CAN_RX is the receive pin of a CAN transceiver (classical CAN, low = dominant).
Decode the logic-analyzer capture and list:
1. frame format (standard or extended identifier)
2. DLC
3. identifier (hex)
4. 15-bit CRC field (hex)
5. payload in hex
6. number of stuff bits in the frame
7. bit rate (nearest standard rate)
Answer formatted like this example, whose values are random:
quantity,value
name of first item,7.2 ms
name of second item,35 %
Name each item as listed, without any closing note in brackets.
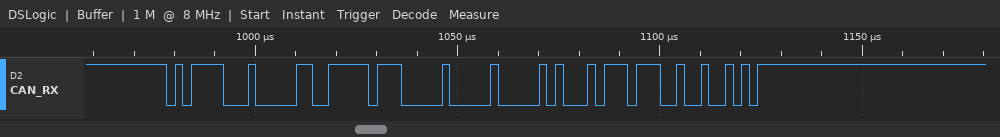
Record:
quantity,value
frame format,standard
DLC,4
identifier,0x5E2
15-bit CRC field,0x5C92
payload in hex,FF 00 00 8B
number of stuff bits in the frame,5
bit rate,500 kbit/s
